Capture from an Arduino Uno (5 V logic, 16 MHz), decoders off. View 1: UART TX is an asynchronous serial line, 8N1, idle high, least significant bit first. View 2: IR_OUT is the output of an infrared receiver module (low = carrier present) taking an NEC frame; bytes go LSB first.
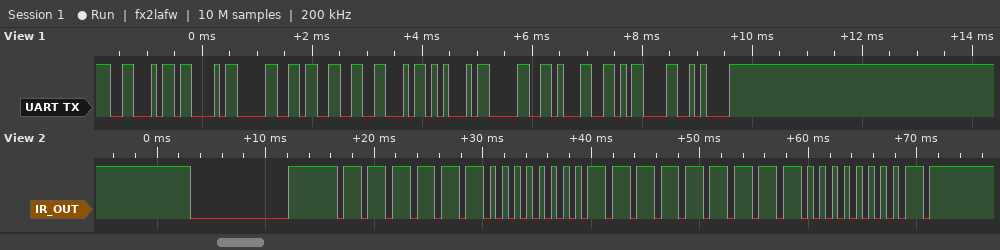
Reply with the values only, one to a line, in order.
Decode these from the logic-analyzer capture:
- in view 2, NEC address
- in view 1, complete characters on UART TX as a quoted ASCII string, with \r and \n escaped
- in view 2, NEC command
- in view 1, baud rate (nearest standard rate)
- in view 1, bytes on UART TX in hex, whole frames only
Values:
0x3F
"FC03FE01\r\n"
0x7F
9600 baud
46 43 30 33 46 45 30 31 0D 0A
